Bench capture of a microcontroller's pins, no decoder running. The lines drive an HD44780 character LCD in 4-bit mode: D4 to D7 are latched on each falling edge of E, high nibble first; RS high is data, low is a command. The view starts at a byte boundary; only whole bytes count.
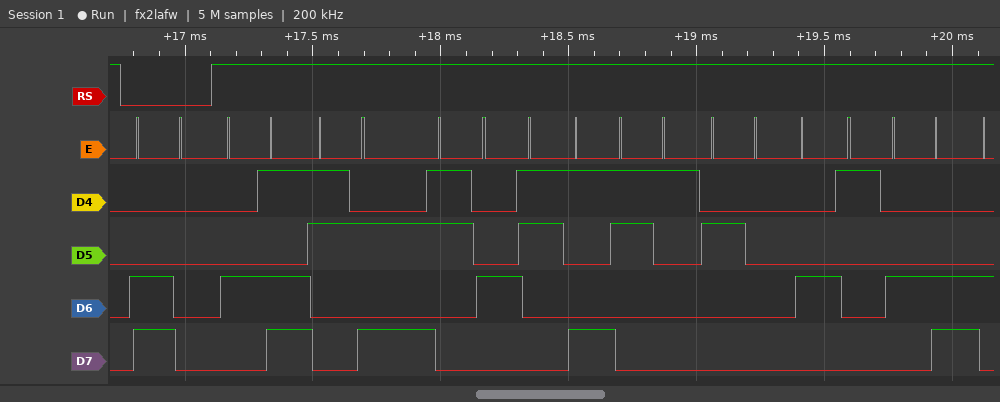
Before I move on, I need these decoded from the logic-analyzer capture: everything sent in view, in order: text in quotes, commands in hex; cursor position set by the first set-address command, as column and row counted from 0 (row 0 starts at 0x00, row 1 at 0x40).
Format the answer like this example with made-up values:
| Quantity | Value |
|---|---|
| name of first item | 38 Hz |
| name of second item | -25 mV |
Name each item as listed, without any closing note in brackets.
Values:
| Quantity | Value |
|---|---|
| everything sent in view, in order: text in quotes, commands in hex | 0xC0 "M:491 AL" |
| cursor position set by the first set-address command, as column and row counted from 0 | column 0, row 1 |
